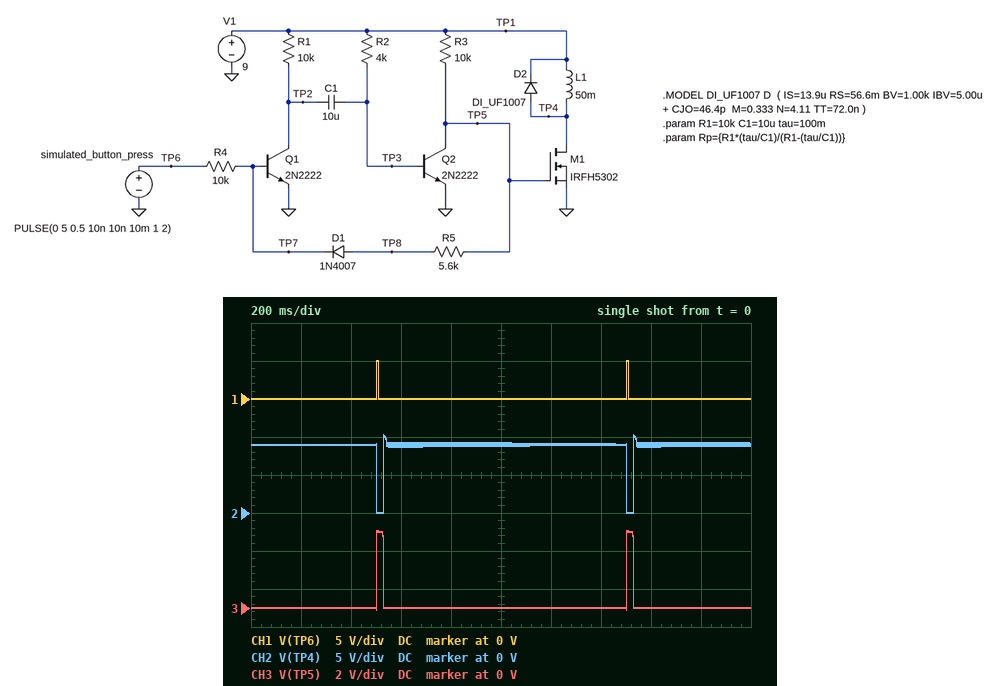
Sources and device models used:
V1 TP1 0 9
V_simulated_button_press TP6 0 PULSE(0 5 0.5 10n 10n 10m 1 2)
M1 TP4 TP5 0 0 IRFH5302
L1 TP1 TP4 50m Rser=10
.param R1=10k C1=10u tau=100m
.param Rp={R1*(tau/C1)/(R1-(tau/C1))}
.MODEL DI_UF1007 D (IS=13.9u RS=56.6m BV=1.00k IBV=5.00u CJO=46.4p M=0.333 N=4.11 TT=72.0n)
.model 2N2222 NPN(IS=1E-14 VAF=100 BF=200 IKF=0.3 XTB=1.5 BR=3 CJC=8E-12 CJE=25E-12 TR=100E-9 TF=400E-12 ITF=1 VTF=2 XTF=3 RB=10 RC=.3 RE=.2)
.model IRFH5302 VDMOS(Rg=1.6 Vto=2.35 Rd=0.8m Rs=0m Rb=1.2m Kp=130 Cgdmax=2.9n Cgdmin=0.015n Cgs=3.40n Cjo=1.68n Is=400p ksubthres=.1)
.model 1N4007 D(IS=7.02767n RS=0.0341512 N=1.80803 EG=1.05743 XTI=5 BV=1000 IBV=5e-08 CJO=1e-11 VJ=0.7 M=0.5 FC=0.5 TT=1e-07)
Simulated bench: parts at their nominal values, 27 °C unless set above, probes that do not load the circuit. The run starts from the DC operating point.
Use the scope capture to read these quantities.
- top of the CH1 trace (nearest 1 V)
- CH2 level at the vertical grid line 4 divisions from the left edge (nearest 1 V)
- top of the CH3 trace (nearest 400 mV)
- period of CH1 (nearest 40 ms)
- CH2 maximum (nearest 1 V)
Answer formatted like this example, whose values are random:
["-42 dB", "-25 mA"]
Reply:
["5 V", "9 V", "4.0 V", "1.00 s", "10 V"]
